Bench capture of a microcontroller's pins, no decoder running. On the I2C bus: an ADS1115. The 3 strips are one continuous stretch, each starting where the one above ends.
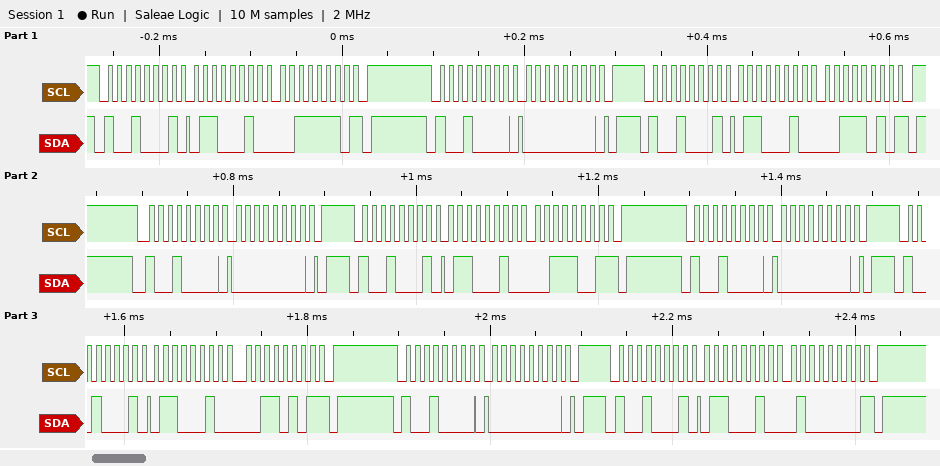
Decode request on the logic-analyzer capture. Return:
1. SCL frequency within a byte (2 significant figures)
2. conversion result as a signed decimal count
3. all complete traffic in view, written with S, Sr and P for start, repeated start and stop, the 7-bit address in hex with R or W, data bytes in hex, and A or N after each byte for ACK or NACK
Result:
100 kHz
25146
S 48R A 62 A 3E N P S 48W A 00 A P S 48R A 62 A 3A N P S 48W A 00 A P S 48R A 62 A 39 N P S 48W A 00 A P S 48R A 62 A 35 N P S 48W A 00 A P S 48R A 62 A 40 N P
